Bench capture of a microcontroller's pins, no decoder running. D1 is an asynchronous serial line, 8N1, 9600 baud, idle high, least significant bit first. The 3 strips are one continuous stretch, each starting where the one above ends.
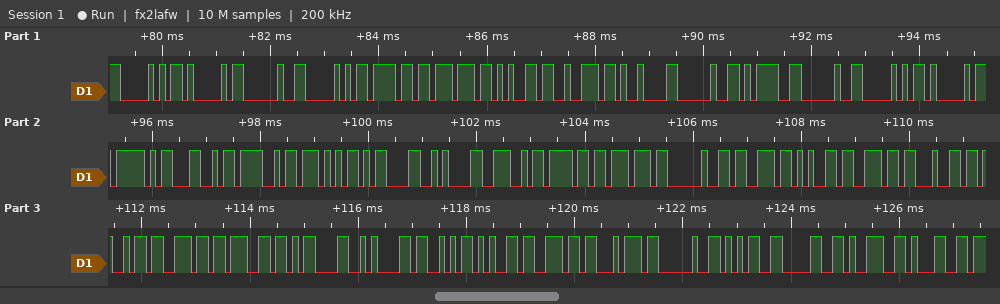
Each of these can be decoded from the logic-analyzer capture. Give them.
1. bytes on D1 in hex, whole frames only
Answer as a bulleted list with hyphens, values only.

- 50 41 20 50 6F 77 65 72 09 20 3D 20 50 41 5F 4C 4F 57 0D 0A 4E 6F 77 20 73 65 6E 64 69 6E 67 0D 0A 53 65 6E 74 20 35 30 39 31
